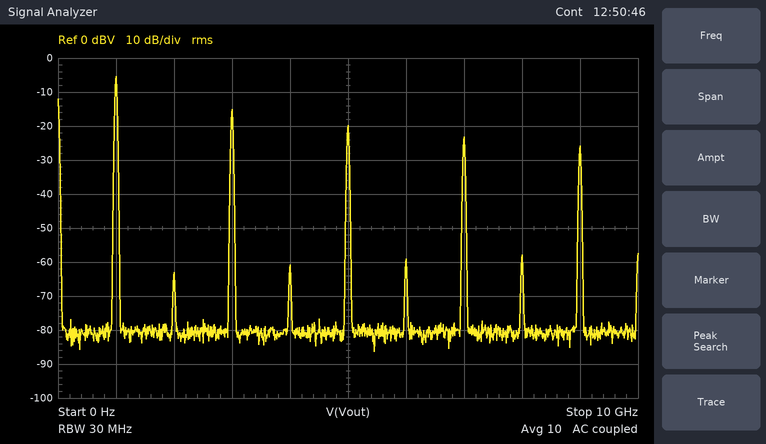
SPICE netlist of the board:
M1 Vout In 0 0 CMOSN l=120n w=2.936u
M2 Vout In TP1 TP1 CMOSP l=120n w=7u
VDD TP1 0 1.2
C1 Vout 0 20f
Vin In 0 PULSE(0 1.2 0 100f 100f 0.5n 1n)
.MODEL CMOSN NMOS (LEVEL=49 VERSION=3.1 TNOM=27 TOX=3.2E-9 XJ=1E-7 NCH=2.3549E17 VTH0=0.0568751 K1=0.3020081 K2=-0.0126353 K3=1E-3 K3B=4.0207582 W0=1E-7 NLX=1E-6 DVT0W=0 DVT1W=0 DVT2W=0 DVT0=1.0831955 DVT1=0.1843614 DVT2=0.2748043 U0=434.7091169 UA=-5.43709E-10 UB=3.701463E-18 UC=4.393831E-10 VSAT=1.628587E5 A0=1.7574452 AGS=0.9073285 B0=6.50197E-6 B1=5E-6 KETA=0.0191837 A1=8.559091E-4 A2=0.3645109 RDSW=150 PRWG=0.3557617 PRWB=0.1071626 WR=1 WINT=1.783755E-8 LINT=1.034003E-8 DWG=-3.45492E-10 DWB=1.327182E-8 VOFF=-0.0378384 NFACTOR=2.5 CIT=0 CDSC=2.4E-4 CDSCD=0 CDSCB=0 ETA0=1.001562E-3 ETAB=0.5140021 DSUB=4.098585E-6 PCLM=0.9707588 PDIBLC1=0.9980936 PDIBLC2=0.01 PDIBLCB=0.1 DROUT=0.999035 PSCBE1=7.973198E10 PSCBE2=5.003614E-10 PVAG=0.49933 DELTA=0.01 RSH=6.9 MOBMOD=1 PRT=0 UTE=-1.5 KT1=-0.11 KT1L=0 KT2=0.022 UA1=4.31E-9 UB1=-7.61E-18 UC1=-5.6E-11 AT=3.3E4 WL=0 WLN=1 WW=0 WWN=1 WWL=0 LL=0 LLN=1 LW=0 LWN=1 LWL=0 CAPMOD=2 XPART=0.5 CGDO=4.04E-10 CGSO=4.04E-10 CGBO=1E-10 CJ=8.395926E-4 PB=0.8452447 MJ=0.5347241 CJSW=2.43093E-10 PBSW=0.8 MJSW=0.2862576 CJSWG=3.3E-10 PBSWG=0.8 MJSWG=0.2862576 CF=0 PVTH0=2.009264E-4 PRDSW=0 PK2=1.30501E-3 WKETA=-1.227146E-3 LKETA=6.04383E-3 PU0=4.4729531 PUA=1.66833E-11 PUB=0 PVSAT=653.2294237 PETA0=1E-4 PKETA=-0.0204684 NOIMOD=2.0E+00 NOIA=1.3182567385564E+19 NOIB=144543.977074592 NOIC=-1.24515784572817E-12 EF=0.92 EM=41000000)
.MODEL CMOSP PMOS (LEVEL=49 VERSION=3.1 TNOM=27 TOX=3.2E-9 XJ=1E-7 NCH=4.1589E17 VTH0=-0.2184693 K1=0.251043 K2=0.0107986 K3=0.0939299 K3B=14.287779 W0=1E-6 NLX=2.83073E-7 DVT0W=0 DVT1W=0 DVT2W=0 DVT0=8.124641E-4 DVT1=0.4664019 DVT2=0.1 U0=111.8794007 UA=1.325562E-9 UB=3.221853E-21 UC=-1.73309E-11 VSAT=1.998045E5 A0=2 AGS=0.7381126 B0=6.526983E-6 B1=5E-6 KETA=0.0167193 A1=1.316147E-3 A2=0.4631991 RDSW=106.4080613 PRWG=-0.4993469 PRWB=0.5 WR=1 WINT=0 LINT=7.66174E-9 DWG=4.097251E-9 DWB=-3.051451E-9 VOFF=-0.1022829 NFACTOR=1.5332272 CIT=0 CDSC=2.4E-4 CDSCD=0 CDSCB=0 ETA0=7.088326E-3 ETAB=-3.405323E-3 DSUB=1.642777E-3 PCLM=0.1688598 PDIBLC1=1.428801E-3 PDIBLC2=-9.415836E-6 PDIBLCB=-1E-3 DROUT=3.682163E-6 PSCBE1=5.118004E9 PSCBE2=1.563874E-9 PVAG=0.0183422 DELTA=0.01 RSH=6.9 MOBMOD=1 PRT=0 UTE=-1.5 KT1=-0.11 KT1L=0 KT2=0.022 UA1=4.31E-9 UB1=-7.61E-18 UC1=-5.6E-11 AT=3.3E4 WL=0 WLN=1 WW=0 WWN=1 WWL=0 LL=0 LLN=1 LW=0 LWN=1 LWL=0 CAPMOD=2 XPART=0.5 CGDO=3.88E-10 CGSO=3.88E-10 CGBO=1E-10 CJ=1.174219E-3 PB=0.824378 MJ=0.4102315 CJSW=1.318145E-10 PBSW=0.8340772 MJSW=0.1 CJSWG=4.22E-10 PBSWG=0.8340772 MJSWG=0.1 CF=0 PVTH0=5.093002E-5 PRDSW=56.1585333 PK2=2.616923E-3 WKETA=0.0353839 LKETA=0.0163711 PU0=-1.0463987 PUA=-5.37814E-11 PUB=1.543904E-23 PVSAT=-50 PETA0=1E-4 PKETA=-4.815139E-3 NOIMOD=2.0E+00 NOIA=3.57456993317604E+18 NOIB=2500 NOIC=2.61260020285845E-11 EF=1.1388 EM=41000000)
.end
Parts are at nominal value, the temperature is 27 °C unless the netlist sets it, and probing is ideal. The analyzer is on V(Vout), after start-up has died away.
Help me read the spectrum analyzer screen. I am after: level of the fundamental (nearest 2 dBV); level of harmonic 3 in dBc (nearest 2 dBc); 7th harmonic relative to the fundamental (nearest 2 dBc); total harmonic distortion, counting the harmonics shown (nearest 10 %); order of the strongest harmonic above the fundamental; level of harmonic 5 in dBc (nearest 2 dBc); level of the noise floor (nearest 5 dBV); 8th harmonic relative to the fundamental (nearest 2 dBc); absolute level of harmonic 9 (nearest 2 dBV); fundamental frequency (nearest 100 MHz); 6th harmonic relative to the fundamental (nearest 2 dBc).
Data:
-6 dBV
-10 dBc
-18 dBc
40 %
3
-14 dBc
-80 dBV
-52 dBc
-26 dBV
1.0 GHz
-54 dBc
